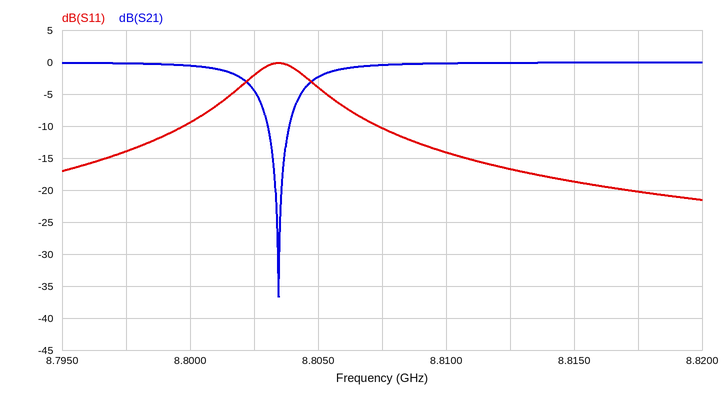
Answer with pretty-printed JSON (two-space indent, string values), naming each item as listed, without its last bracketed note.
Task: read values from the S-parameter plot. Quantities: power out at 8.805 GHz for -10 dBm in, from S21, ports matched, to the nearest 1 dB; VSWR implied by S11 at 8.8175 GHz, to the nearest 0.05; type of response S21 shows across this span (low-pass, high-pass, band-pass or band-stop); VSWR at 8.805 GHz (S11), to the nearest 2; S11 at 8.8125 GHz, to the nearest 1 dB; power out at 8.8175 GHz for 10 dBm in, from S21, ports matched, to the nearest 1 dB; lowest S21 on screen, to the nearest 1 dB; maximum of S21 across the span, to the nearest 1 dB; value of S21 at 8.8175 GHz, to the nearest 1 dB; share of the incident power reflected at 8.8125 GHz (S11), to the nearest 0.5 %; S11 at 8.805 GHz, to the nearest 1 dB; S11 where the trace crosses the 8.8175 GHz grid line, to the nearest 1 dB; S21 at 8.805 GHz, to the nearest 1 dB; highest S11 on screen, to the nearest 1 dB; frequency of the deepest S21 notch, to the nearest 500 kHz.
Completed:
{
  "power out at 8.805 GHz for -10 dBm in, from S21, ports matched, to the nearest 1 dB": "-12 dBm",
  "VSWR implied by S11 at 8.8175 GHz, to the nearest 0.05": "1.20",
  "type of response S21 shows across this span": "band-stop",
  "VSWR at 8.805 GHz (S11), to the nearest 2": "4",
  "S11 at 8.8125 GHz, to the nearest 1 dB": "-17 dB",
  "power out at 8.8175 GHz for 10 dBm in, from S21, ports matched, to the nearest 1 dB": "10 dBm",
  "lowest S21 on screen, to the nearest 1 dB": "-37 dB",
  "maximum of S21 across the span, to the nearest 1 dB": "0 dB",
  "value of S21 at 8.8175 GHz, to the nearest 1 dB": "0 dB",
  "share of the incident power reflected at 8.8125 GHz (S11), to the nearest 0.5 %": "2.0 %",
  "S11 at 8.805 GHz, to the nearest 1 dB": "-4 dB",
  "S11 where the trace crosses the 8.8175 GHz grid line, to the nearest 1 dB": "-20 dB",
  "S21 at 8.805 GHz, to the nearest 1 dB": "-2 dB",
  "highest S11 on screen, to the nearest 1 dB": "0 dB",
  "frequency of the deepest S21 notch, to the nearest 500 kHz": "8.8035 GHz"
}
